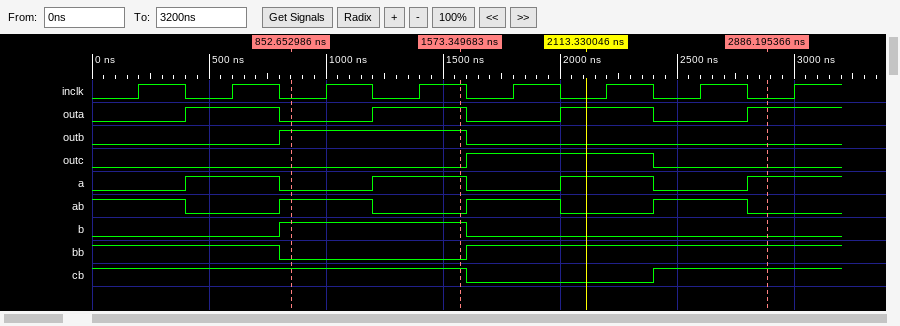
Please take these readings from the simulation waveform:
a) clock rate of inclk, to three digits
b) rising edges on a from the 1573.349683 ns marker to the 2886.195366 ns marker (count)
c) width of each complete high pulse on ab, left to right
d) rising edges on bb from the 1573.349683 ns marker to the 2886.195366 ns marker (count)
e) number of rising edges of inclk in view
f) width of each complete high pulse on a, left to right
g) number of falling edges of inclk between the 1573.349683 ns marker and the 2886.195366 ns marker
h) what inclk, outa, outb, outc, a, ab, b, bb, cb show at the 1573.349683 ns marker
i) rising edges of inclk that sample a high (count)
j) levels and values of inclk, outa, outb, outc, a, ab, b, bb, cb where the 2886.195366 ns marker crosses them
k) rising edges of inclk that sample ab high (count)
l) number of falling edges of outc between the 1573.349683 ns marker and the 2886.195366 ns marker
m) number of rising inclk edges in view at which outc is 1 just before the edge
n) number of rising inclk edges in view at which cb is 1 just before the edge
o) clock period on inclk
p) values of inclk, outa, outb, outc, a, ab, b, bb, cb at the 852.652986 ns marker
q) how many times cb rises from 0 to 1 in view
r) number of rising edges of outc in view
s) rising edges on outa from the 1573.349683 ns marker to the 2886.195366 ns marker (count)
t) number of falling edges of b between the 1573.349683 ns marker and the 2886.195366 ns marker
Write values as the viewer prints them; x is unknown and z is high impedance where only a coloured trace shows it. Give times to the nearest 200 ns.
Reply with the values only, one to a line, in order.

2.50 MHz
2
400 ns, 400 ns, 400 ns
1
8
400 ns, 400 ns, 400 ns
4
inclk=1, outa=1, outb=1, outc=0, a=1, ab=0, b=1, bb=0, cb=1
4
inclk=0, outa=1, outb=0, outc=0, a=1, ab=0, b=0, bb=1, cb=1
4
1
2
6
400 ns
inclk=0, outa=0, outb=1, outc=0, a=0, ab=1, b=1, bb=0, cb=1
1
1
2
1
